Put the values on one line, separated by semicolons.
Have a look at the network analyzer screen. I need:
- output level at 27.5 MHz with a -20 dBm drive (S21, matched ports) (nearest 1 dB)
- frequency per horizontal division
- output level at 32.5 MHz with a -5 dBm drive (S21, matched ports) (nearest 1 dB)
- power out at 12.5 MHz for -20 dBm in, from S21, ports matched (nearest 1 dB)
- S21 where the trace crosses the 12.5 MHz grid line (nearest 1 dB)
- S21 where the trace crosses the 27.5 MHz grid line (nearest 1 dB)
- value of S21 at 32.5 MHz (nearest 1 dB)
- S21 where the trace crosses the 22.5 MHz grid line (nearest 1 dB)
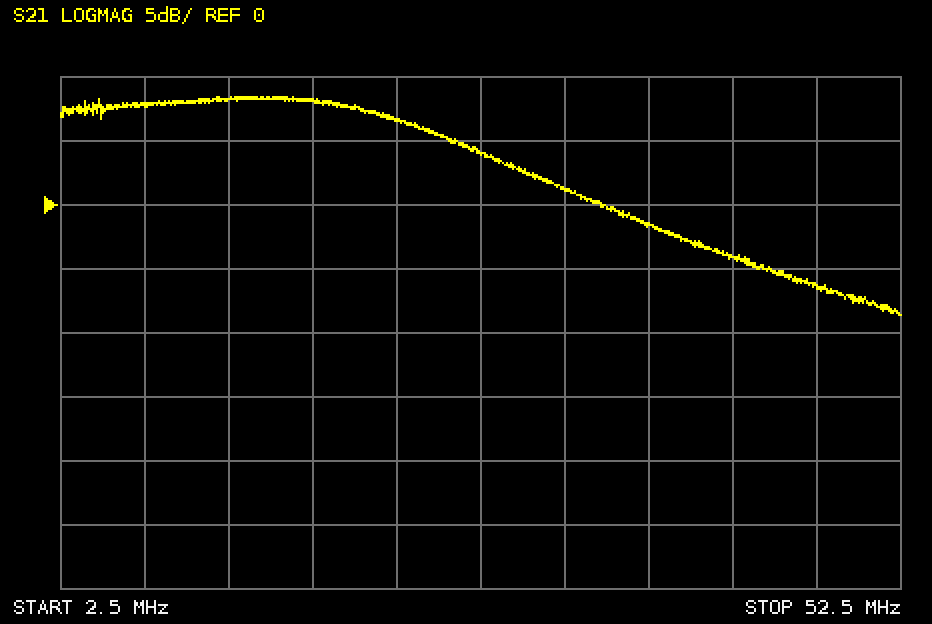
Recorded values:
-16 dBm; 5 MHz; -4 dBm; -12 dBm; 8 dB; 4 dB; 1 dB; 7 dB
